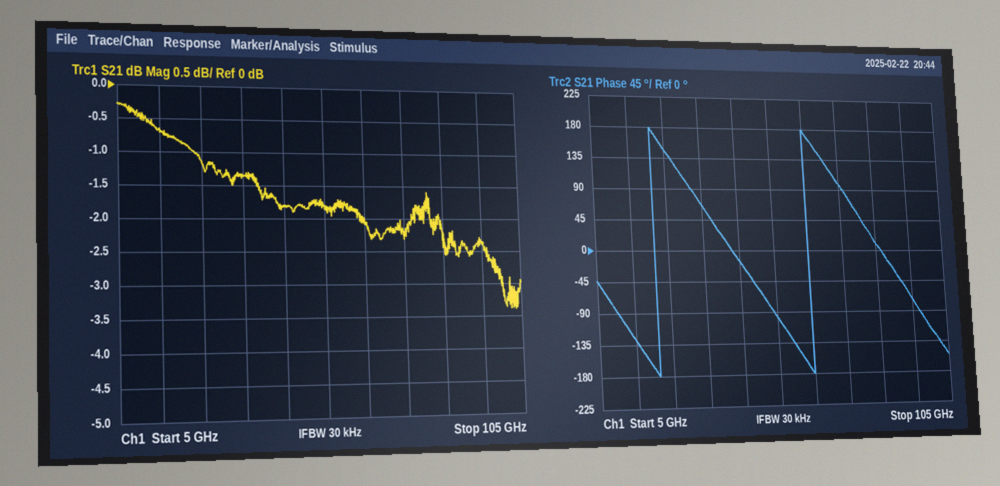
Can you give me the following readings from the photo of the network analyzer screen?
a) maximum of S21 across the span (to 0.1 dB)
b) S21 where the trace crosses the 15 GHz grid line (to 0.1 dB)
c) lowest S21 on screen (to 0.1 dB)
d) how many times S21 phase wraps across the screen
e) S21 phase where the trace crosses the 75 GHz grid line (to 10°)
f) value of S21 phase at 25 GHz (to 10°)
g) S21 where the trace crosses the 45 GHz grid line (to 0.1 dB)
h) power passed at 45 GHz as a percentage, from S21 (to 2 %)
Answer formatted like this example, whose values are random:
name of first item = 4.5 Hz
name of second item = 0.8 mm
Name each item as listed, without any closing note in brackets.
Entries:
maximum of S21 across the span = -0.3 dB
S21 where the trace crosses the 15 GHz grid line = -0.7 dB
lowest S21 on screen = -3.4 dB
how many times S21 phase wraps across the screen = 2
S21 phase where the trace crosses the 75 GHz grid line = 100°
value of S21 phase at 25 GHz = 150°
S21 where the trace crosses the 45 GHz grid line = -1.8 dB
power passed at 45 GHz as a percentage, from S21 = 66 %
